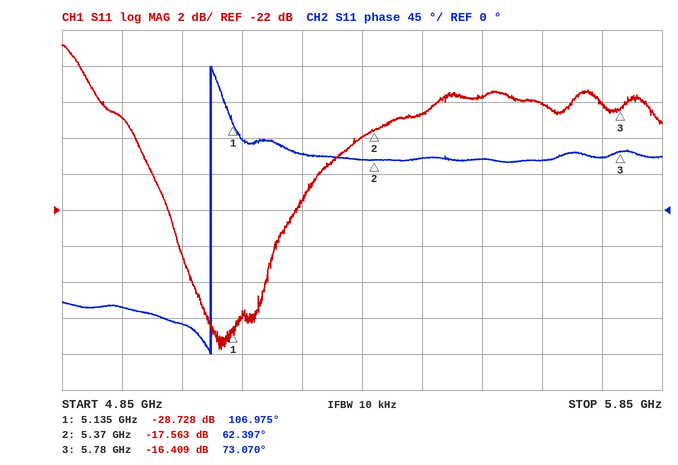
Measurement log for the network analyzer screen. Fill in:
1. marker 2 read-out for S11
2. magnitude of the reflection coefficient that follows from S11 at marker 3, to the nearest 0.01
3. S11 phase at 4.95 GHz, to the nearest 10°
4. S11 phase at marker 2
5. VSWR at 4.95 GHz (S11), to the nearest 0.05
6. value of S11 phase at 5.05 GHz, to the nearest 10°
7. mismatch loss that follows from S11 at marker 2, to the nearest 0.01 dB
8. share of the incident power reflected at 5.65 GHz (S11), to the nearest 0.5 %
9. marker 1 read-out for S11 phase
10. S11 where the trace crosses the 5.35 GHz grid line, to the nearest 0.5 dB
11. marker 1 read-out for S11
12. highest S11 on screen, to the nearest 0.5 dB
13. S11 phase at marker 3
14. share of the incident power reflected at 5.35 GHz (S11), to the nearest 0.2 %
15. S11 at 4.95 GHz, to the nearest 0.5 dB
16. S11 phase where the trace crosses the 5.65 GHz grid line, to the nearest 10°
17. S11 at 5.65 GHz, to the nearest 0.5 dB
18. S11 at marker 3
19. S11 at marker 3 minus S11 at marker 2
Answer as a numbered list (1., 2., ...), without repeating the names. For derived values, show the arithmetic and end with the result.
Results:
1. -17.563 dB
2. 10^(-16.409/20) ≈ 0.15
3. -120°
4. 62.397°
5. |Γ| = 10^(-17/20) = 0.1413; VSWR = (1 + 0.1413)/(1 − 0.1413) ≈ 1.33, so 1.35 to the nearest 0.05
6. -140°
7. −10 log10(1 − 10^(-17.563/10)) ≈ 0.08 dB
8. 10^(-16/10) ≈ 2.5 %
9. 106.975°
10. -18.0 dB
11. -28.728 dB
12. -13.0 dB
13. 73.070°
14. 10^(-18/10) ≈ 1.6 %
15. -17.0 dB
16. 60°
17. -16.0 dB
18. -16.409 dB
19. -16.409 − (-17.563) = 1.154 dB
